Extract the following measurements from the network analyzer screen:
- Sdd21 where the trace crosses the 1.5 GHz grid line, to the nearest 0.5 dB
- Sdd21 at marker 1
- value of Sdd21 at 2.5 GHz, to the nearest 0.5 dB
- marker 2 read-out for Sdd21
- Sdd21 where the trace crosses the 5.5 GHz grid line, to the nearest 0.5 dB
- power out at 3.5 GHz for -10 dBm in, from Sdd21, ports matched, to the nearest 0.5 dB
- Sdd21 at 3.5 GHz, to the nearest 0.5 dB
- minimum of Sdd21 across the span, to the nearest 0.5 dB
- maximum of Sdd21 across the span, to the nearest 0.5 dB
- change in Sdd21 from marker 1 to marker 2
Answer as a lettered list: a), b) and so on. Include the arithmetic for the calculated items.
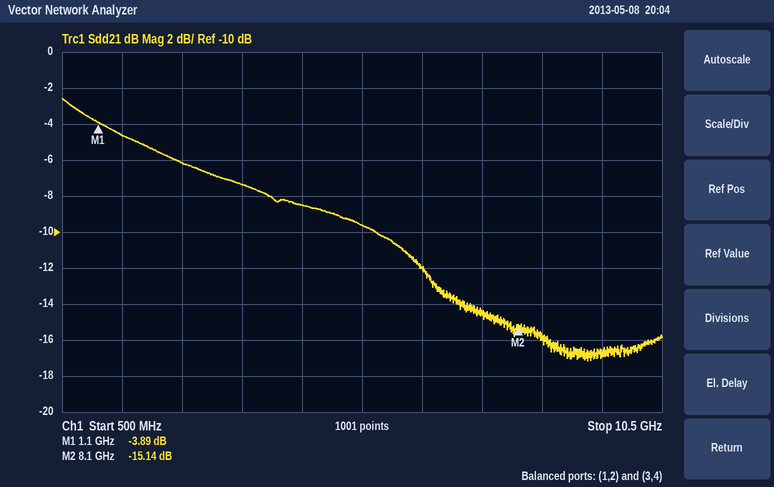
a) -4.5 dB
b) -3.89 dB
c) -6.0 dB
d) -15.14 dB
e) -9.5 dB
f) -10 dBm + (-7.5 dB) = -17.5 dBm
g) -7.5 dB
h) -17.0 dB
i) -2.5 dB
j) -15.14 − (-3.89) = -11.25 dB
